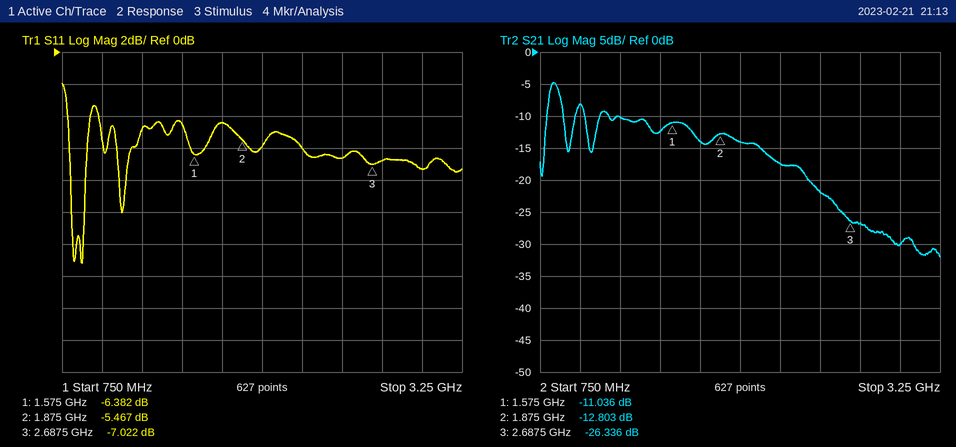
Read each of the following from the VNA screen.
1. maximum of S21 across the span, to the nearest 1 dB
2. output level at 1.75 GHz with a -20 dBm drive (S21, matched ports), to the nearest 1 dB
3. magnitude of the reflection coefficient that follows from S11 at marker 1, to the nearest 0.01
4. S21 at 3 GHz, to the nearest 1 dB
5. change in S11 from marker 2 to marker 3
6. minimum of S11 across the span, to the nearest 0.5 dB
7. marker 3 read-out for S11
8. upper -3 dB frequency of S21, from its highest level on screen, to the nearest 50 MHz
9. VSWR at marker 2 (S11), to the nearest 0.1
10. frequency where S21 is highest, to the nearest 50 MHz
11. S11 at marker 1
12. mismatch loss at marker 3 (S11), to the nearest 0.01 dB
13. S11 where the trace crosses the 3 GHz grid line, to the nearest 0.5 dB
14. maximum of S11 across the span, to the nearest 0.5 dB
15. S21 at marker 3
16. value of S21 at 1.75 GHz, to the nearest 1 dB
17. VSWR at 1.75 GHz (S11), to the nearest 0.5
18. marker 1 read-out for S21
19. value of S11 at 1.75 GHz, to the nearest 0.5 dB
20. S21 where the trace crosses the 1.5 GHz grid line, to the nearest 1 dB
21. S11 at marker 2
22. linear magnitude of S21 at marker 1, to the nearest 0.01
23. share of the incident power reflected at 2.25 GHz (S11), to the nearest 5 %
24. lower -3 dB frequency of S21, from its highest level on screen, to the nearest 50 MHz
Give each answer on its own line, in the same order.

-5 dB
-34 dBm
0.48
-30 dB
-1.555 dB
-13.0 dB
-7.022 dB
900 MHz
3.3
850 MHz
-6.382 dB
0.96 dB
-7.5 dB
-2.0 dB
-26.336 dB
-14 dB
4.0
-11.036 dB
-4.5 dB
-12 dB
-5.467 dB
0.28
25 %
800 MHz
